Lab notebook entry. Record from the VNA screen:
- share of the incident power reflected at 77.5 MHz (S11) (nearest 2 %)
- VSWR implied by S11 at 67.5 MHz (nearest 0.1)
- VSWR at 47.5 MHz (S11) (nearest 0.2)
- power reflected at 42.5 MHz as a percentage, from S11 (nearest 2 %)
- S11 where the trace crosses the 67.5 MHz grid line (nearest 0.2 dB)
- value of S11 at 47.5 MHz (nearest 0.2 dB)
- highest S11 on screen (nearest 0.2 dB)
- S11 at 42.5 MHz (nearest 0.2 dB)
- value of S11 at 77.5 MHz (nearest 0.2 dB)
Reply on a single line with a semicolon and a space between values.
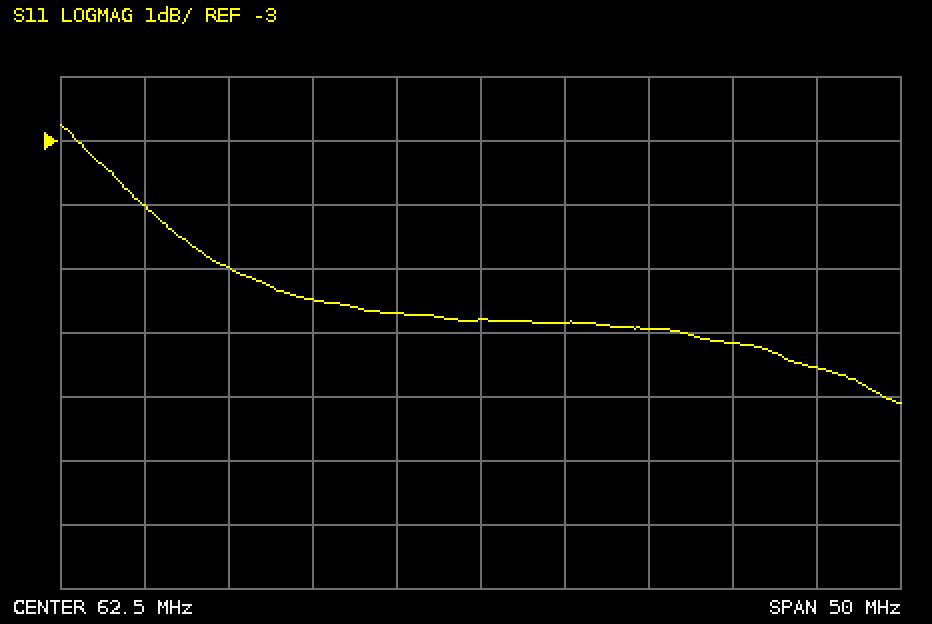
24 %; 3.1; 3.6; 40 %; -5.8 dB; -5.0 dB; -2.8 dB; -4.0 dB; -6.2 dB
